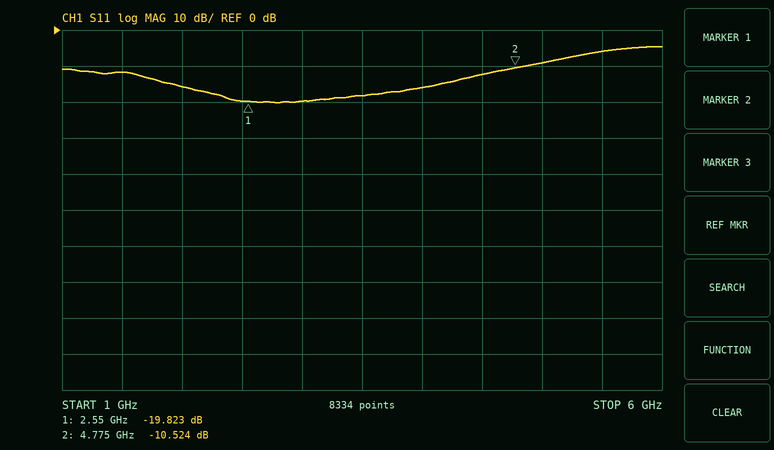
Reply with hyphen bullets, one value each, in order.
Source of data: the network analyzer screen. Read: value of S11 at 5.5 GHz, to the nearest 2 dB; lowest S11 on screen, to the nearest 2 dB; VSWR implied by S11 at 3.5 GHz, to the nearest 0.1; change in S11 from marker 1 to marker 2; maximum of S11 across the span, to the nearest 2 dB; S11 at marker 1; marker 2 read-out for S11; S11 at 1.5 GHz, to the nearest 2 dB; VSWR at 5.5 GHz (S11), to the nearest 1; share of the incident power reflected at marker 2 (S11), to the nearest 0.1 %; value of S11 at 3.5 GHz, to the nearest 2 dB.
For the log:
- -6 dB
- -20 dB
- 1.3
- 9.299 dB
- -4 dB
- -19.823 dB
- -10.524 dB
- -12 dB
- 3
- 8.9 %
- -18 dB
